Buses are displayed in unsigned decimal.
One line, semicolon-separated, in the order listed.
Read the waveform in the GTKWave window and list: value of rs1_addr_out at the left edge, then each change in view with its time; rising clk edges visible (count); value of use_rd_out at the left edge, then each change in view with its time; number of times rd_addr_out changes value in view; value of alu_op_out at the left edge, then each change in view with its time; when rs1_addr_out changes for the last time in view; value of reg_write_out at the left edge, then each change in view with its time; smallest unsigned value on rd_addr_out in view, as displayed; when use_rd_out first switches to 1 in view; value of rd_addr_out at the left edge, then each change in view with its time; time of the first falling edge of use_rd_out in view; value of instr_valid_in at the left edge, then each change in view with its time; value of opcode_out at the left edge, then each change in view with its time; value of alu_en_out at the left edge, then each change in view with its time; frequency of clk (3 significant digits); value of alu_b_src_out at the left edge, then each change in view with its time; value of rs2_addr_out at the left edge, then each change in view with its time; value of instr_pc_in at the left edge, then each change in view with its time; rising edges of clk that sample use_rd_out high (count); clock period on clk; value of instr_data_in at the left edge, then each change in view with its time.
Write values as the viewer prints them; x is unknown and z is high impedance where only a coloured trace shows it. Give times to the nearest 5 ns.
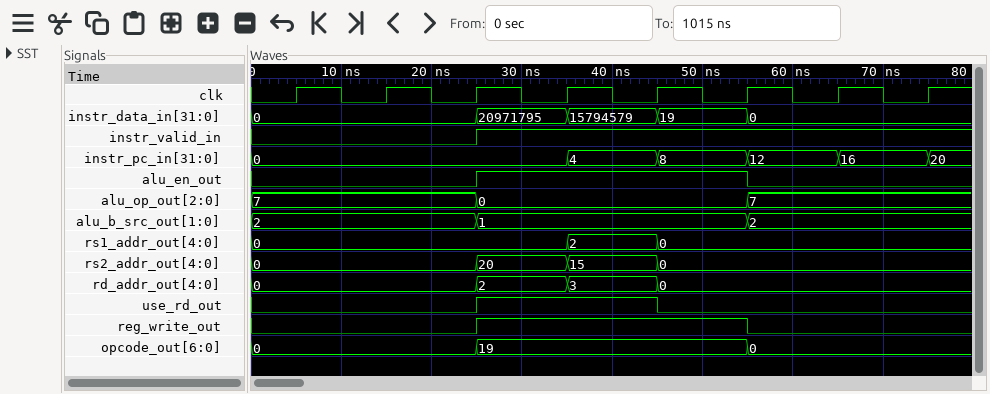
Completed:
0, 2 at 35 ns, 0 at 45 ns; 8; 0, 1 at 25 ns, 0 at 45 ns; 3; 7, 0 at 25 ns, 7 at 55 ns; 45 ns; 0, 1 at 25 ns, 0 at 55 ns; 0; 25 ns; 0, 2 at 25 ns, 3 at 35 ns, 0 at 45 ns; 45 ns; 0, 1 at 25 ns; 0, 19 at 25 ns, 0 at 55 ns; 0, 1 at 25 ns, 0 at 55 ns; 100 MHz; 2, 1 at 25 ns, 2 at 55 ns; 0, 20 at 25 ns, 15 at 35 ns, 0 at 45 ns; 0, 4 at 35 ns, 8 at 45 ns, 12 at 55 ns, 16 at 65 ns, 20 at 75 ns; 2; 10 ns; 0, 20971795 at 25 ns, 15794579 at 35 ns, 19 at 45 ns, 0 at 55 ns
